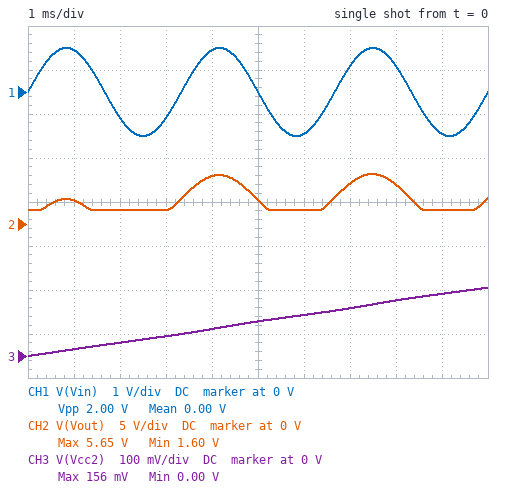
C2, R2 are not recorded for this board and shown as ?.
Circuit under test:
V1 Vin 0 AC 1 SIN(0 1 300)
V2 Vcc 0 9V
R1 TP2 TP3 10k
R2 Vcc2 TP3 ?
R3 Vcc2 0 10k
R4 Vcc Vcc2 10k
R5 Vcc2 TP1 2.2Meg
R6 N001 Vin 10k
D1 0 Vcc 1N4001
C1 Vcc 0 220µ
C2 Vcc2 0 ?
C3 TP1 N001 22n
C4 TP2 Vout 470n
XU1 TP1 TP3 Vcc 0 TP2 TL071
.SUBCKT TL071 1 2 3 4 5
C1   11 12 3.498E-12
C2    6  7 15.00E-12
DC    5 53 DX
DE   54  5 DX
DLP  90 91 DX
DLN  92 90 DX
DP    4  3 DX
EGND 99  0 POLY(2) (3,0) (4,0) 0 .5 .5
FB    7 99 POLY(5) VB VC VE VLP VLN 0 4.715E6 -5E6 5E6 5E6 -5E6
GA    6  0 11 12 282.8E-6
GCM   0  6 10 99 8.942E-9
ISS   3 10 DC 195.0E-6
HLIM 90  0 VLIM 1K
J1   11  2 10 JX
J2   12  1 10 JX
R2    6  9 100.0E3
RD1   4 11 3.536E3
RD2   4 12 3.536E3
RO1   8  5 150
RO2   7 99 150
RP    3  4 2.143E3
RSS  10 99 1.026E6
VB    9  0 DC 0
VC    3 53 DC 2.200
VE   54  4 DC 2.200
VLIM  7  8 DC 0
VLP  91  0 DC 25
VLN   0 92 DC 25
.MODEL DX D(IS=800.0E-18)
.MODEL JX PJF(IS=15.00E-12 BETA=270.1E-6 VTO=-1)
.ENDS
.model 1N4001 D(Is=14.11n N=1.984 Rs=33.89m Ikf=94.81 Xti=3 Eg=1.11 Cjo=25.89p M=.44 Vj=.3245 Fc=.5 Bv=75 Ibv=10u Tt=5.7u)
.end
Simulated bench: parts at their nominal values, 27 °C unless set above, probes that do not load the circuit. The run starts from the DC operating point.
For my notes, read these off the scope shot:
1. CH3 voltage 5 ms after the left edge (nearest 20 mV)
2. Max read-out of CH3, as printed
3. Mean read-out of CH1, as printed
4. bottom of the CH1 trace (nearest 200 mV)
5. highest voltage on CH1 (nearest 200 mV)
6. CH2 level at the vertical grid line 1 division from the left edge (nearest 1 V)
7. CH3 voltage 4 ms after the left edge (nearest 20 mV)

80 mV
156 mV
0.00 V
-1.0 V
1.0 V
3 V
60 mV
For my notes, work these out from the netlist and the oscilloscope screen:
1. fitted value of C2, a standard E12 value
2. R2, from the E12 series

68 µF
5.6 kΩ
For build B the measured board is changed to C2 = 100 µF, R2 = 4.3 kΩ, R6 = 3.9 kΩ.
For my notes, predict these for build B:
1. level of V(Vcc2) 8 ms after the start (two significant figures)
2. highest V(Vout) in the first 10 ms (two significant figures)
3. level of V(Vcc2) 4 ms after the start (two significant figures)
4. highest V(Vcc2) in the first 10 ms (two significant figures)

91 mV
6.9 V
43 mV
110 mV
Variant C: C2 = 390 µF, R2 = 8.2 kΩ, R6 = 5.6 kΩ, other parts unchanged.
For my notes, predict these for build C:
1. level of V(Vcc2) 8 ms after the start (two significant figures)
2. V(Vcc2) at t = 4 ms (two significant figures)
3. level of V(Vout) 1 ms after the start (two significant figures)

21 mV
10 mV
2.2 V
